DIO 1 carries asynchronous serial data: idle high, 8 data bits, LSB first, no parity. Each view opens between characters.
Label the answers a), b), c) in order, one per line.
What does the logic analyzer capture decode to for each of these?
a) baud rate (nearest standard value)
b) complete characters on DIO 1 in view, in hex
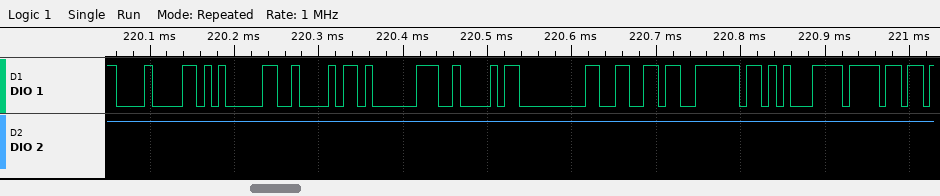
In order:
a) 115200 baud
b) 08, 05, 42, 81, 42, 00, 66, 7E, C5, 6F
